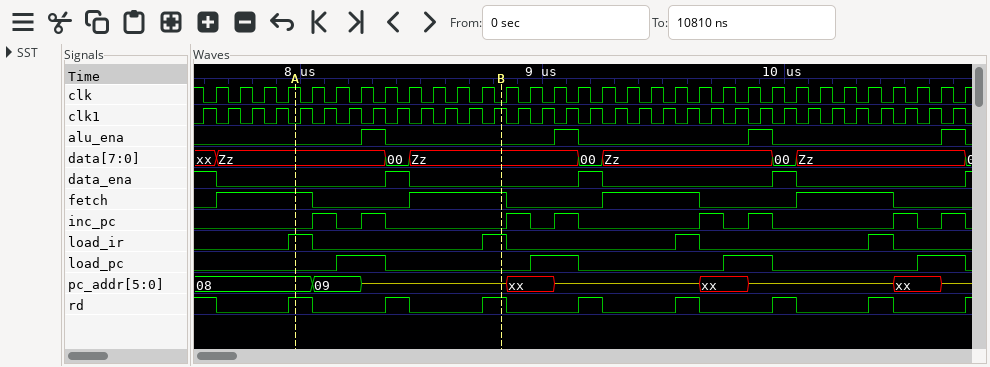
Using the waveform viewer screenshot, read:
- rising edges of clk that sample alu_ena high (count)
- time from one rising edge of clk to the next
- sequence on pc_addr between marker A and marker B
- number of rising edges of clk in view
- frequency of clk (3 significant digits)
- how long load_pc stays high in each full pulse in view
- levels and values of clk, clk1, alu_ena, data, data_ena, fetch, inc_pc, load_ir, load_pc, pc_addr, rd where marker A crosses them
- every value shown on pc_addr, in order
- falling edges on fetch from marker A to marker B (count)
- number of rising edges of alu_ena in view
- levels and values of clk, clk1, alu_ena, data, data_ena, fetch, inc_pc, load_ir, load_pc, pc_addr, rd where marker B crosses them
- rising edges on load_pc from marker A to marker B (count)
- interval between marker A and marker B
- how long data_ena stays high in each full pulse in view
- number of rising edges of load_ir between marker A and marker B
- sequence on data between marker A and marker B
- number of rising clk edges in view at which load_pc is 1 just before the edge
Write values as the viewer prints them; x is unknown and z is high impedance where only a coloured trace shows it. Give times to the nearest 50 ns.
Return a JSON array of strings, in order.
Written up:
["4", "100 ns", "08, 09, z", "32", "10.0 MHz", "200 ns, 200 ns, 200 ns, 200 ns", "clk=1, clk1=0, alu_ena=0, data=Zz, data_ena=0, fetch=1, inc_pc=0, load_ir=1, load_pc=0, pc_addr=08, rd=1", "08, 09, z, xx, z, xx, z, xx, z", "1", "4", "clk=0, clk1=1, alu_ena=0, data=Zz, data_ena=0, fetch=1, inc_pc=0, load_ir=1, load_pc=0, pc_addr=z, rd=1", "1", "850 ns", "100 ns, 100 ns, 100 ns", "1", "Zz, 00, Zz", "8"]
